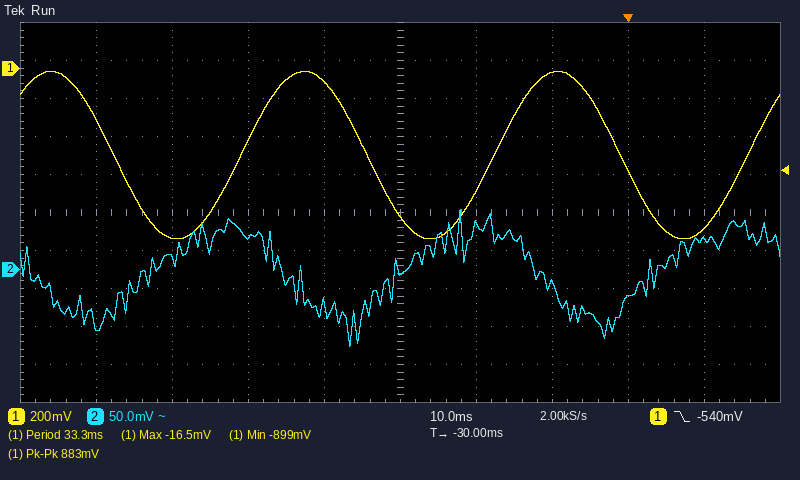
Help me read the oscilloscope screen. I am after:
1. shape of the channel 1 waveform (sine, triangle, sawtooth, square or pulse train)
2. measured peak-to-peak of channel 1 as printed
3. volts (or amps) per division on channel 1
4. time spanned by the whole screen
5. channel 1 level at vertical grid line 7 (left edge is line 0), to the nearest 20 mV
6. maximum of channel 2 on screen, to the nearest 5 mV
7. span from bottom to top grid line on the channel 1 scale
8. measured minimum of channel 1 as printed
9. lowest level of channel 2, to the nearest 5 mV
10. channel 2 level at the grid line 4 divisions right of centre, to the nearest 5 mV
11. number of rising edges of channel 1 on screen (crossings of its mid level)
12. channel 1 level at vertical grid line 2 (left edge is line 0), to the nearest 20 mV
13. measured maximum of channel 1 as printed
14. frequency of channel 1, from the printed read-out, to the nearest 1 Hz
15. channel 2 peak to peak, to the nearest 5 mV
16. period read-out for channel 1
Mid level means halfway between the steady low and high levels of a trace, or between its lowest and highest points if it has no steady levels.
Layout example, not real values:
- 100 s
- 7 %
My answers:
- sine
- 883 mV
- 200 mV
- 100 ms
- -20 mV
- 80 mV
- 2 V
- -899 mV
- -100 mV
- 40 mV
- 3
- -900 mV
- -16.5 mV
- 30 Hz
- 180 mV
- 33.3 ms
